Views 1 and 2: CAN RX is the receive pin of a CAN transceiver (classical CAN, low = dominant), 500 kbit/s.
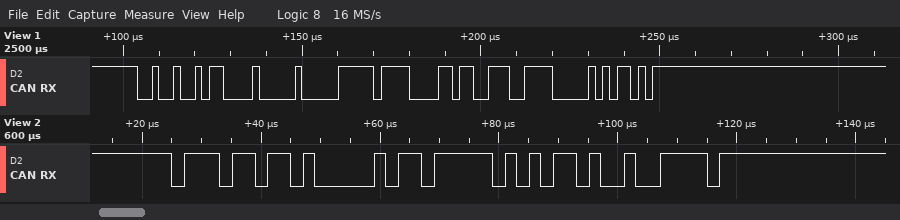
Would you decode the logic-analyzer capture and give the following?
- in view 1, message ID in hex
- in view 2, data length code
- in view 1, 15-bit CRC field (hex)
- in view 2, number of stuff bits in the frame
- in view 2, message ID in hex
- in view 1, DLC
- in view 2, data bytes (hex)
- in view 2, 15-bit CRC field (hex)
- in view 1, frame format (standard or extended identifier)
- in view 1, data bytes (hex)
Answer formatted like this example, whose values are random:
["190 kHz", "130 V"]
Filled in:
["0x24B", "1", "0x7816", "2", "0x76D", "4", "BF", "0x2D27", "standard", "00 FF 0D 9C"]
